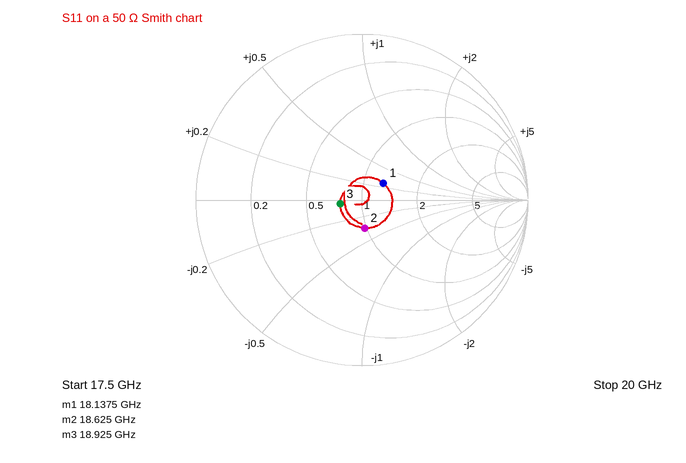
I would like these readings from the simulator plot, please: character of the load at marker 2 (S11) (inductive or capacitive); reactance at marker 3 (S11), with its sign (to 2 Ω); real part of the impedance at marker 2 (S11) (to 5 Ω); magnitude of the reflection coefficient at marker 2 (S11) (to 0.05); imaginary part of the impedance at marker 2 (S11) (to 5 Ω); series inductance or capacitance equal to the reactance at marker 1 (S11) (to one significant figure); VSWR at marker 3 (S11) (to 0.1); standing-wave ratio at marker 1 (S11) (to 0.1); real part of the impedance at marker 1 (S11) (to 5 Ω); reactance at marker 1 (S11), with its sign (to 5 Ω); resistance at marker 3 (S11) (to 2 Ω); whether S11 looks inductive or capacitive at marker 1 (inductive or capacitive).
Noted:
capacitive
-2 Ω
50 Ω
0.15
-15 Ω
100 pH
1.3
1.4
65 Ω
+15 Ω
38 Ω
inductive
